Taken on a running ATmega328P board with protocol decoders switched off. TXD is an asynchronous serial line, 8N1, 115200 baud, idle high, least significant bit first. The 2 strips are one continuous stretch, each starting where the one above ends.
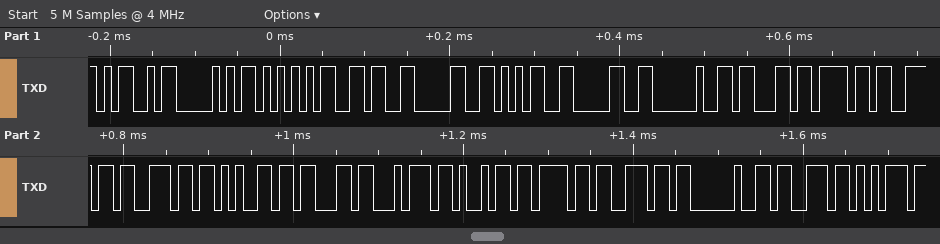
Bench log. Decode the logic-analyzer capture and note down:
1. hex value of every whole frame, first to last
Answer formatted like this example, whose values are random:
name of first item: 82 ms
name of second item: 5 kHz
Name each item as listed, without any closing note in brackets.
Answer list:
hex value of every whole frame, first to last: 0x4D 0x50 0x55 0x36 0x30 0x35 0x30 0x20 0x63 0x6F 0x6E 0x6E 0x65 0x63 0x74 0x69 0x6F 0x6E 0x20 0x73 0x75
